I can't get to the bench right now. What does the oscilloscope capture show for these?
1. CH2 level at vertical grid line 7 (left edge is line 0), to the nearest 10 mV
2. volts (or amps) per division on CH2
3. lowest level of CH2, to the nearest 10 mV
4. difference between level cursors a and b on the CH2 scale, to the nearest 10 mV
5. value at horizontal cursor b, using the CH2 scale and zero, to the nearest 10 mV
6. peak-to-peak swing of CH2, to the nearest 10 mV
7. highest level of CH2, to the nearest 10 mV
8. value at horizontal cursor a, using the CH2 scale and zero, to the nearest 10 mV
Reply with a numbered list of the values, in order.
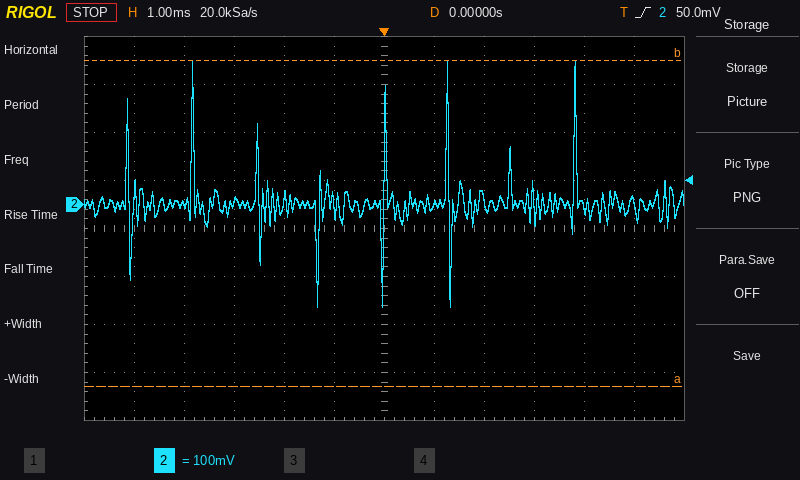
1. 0 mV
2. 100 mV
3. -210 mV
4. 680 mV
5. 300 mV
6. 510 mV
7. 300 mV
8. -380 mV
